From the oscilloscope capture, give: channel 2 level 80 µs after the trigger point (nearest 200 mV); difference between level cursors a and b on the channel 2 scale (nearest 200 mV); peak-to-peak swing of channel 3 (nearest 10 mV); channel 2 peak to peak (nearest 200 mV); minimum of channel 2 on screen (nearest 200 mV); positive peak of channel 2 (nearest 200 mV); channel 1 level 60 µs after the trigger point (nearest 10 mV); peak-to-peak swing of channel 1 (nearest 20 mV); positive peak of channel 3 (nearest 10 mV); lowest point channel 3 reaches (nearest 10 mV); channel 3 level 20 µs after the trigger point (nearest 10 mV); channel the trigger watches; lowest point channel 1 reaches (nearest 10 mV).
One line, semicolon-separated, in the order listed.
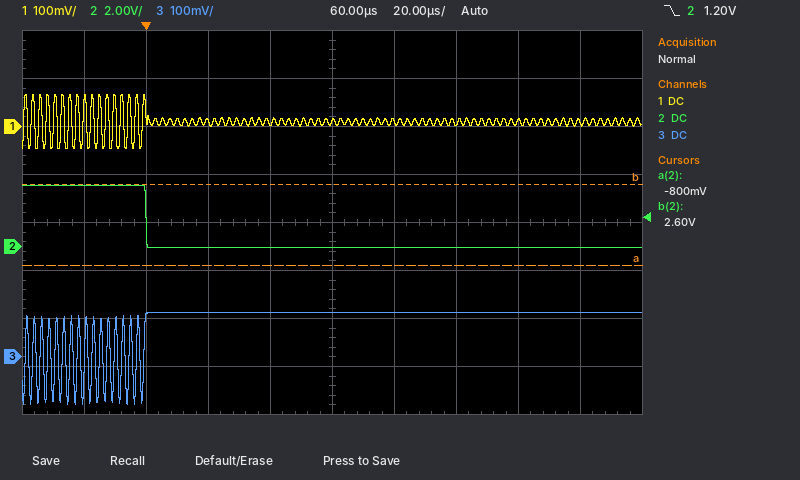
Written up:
0.0 V; 3.4 V; 190 mV; 2.6 V; 0.0 V; 2.6 V; 10 mV; 120 mV; 90 mV; -100 mV; 90 mV; channel 2; -50 mV
